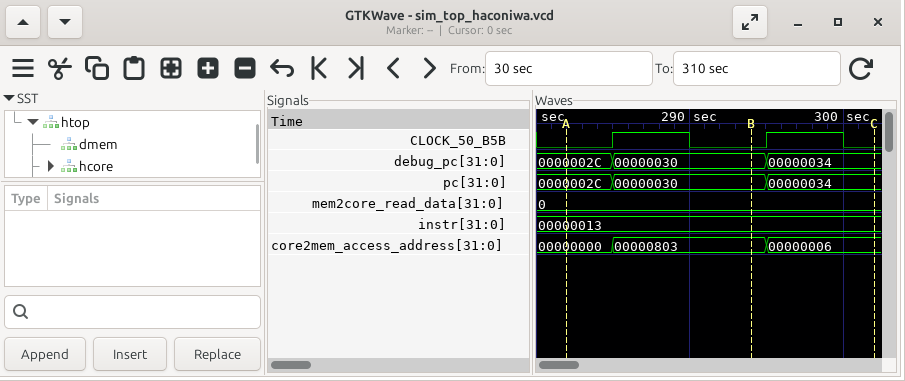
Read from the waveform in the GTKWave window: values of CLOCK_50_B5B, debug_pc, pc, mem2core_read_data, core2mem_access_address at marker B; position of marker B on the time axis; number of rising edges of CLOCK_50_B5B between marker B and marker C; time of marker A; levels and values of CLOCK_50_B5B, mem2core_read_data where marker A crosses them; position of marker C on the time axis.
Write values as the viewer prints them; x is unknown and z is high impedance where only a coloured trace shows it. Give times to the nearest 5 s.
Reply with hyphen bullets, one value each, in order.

- CLOCK_50_B5B=0, debug_pc=00000030, pc=00000030, mem2core_read_data=0, core2mem_access_address=00000803
- 295 s
- 1
- 280 s
- CLOCK_50_B5B=0, mem2core_read_data=0
- 300 s
